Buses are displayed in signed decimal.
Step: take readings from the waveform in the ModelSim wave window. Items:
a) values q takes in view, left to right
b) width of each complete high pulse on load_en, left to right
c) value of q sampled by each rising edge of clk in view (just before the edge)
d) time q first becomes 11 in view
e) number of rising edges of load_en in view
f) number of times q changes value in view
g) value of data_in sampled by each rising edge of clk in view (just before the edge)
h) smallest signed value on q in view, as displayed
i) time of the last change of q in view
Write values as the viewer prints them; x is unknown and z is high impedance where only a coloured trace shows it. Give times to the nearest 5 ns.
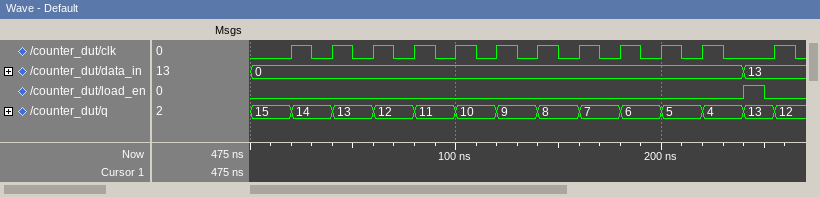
15, 14, 13, 12, 11, 10, 9, 8, 7, 6, 5, 4, 13, 12
10 ns
15, 14, 13, 12, 11, 10, 9, 8, 7, 6, 5, 13
80 ns
1
13
0, 0, 0, 0, 0, 0, 0, 0, 0, 0, 0, 13
4
255 ns
